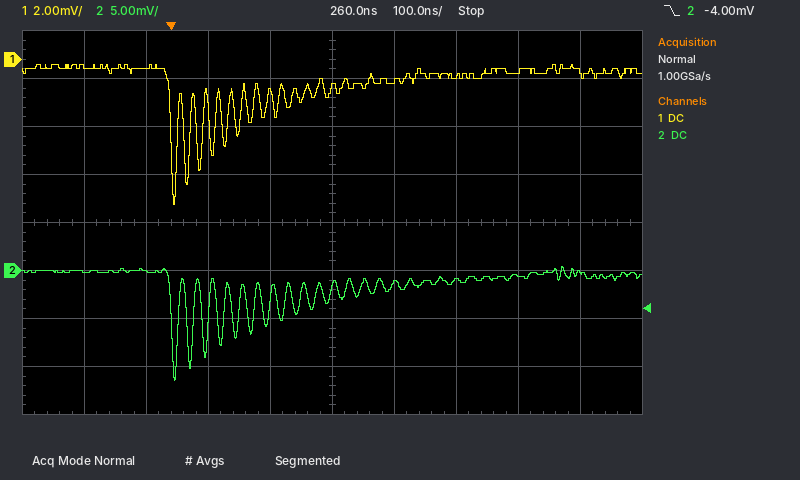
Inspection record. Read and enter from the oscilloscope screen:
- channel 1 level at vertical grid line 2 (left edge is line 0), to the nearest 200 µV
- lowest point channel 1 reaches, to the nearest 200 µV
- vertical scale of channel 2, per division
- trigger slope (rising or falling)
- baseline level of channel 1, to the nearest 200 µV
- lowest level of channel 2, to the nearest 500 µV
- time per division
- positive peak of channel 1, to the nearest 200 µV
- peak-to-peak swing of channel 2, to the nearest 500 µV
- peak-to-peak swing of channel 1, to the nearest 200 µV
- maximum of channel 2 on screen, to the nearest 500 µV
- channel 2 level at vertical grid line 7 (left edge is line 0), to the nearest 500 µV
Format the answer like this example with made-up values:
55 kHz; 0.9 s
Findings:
-400 µV; -6.0 mV; 5 mV; falling; -600 µV; -11.5 mV; 100 ns; -200 µV; 12.0 mV; 5.8 mV; 500 µV; -1.0 mV
